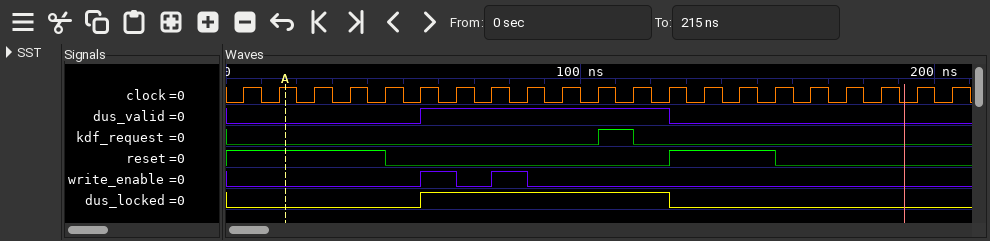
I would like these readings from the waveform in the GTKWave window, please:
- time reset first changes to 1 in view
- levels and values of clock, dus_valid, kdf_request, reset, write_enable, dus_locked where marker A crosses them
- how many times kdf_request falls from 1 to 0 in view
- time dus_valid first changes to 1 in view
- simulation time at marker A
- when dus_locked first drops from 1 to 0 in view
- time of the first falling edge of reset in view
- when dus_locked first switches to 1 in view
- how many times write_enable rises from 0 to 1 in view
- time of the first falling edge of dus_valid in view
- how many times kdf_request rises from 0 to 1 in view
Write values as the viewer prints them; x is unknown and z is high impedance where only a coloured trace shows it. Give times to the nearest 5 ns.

125 ns
clock=1, dus_valid=0, kdf_request=0, reset=1, write_enable=0, dus_locked=0
1
55 ns
15 ns
125 ns
45 ns
55 ns
2
125 ns
1
